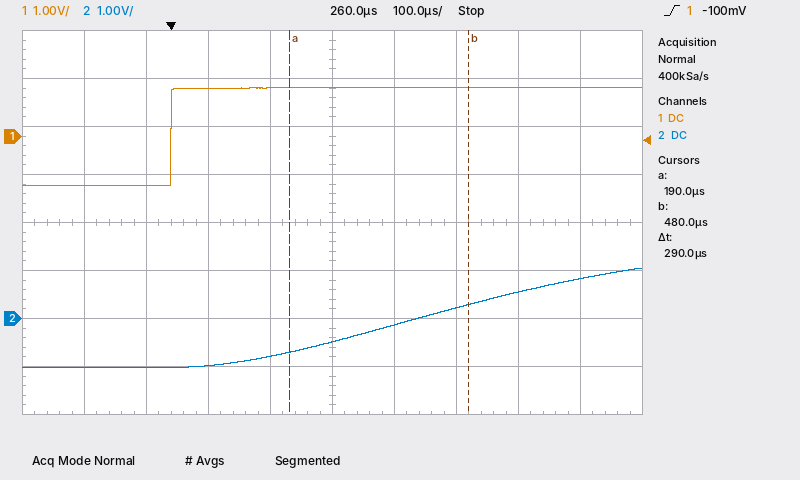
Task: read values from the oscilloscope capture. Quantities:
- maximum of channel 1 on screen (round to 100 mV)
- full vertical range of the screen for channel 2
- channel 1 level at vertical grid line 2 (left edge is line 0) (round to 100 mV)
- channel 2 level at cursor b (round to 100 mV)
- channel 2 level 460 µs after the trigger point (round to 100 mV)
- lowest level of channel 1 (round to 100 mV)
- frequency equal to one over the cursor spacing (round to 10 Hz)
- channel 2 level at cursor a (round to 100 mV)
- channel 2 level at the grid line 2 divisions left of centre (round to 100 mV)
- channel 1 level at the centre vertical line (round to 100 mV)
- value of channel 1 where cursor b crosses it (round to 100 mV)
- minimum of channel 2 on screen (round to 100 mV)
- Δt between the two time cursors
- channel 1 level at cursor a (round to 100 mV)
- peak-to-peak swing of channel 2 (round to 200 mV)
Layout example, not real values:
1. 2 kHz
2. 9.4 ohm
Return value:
1. 1.0 V
2. 8 V
3. -1.0 V
4. 300 mV
5. 200 mV
6. -1.0 V
7. 3.45 kHz
8. -700 mV
9. -1.0 V
10. 1.0 V
11. 1.0 V
12. -1.0 V
13. 290 µs
14. 1.0 V
15. 2.0 V
